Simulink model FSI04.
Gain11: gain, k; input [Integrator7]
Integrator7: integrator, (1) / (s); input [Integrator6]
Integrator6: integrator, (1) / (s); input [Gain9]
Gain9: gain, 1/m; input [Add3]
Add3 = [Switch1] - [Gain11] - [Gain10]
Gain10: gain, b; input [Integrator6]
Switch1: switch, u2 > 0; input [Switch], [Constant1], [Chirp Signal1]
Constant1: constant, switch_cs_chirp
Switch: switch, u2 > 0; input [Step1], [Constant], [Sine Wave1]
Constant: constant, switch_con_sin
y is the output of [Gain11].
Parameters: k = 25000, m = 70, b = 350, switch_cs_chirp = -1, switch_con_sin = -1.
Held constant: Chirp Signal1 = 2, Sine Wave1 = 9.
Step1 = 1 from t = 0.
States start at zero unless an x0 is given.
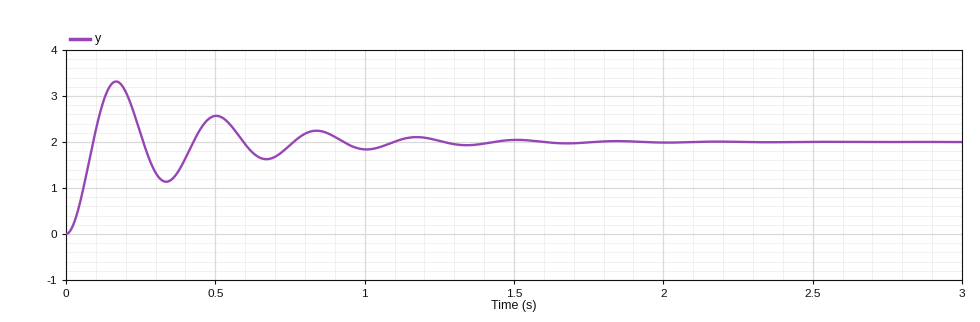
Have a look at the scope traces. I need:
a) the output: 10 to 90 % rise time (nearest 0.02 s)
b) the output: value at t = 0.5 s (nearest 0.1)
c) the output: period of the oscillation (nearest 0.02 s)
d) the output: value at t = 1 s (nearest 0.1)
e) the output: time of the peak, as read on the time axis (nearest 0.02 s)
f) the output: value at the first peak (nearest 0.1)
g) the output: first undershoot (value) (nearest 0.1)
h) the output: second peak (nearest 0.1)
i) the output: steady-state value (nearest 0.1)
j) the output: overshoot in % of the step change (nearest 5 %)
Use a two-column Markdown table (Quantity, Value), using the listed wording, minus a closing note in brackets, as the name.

| Quantity | Value |
|---|---|
| the output: 10 to 90 % rise time | 0.06 s |
| the output: value at t = 0.5 s | 2.6 |
| the output: period of the oscillation | 0.34 s |
| the output: value at t = 1 s | 1.8 |
| the output: time of the peak, as read on the time axis | 0.16 s |
| the output: value at the first peak | 3.3 |
| the output: first undershoot (value) | 1.1 |
| the output: second peak | 2.6 |
| the output: steady-state value | 2.0 |
| the output: overshoot in % of the step change | 65 % |
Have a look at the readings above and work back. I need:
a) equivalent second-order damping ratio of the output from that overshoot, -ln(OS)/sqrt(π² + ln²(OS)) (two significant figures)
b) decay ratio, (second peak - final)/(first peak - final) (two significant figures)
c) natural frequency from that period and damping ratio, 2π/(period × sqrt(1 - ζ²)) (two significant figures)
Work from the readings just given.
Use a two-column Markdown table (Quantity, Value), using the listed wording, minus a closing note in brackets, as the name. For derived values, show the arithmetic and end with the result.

| Quantity | Value |
|---|---|
| equivalent second-order damping ratio of the output from that overshoot, -ln(OS)/sqrt(π² + ln²(OS)) | ln(0.65) = -0.431; 0.431 / sqrt(9.870 + 0.186) = 0.14 |
| decay ratio, (second peak - final)/(first peak - final) | (2.6 - 2) / (3.3 - 2) = 0.46 |
| natural frequency from that period and damping ratio, 2π/(period × sqrt(1 - ζ²)) | 2π / (0.34 × sqrt(1 - 0.14²)) = 19 rad/s |
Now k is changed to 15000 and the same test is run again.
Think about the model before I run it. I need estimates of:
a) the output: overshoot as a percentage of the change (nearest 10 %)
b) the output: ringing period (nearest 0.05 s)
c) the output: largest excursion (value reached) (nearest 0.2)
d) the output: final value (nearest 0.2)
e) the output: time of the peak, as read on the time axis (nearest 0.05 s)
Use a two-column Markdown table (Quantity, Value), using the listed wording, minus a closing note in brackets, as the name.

| Quantity | Value |
|---|---|
| the output: overshoot as a percentage of the change | 60 % |
| the output: ringing period | 0.45 s |
| the output: largest excursion (value reached) | 3.2 |
| the output: final value | 2.0 |
| the output: time of the peak, as read on the time axis | 0.20 s |
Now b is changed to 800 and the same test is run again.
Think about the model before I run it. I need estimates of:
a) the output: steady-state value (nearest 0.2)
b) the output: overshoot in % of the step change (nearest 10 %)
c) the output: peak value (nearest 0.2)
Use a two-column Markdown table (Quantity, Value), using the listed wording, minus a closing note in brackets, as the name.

| Quantity | Value |
|---|---|
| the output: steady-state value | 2.0 |
| the output: overshoot in % of the step change | 40 % |
| the output: peak value | 2.8 |
